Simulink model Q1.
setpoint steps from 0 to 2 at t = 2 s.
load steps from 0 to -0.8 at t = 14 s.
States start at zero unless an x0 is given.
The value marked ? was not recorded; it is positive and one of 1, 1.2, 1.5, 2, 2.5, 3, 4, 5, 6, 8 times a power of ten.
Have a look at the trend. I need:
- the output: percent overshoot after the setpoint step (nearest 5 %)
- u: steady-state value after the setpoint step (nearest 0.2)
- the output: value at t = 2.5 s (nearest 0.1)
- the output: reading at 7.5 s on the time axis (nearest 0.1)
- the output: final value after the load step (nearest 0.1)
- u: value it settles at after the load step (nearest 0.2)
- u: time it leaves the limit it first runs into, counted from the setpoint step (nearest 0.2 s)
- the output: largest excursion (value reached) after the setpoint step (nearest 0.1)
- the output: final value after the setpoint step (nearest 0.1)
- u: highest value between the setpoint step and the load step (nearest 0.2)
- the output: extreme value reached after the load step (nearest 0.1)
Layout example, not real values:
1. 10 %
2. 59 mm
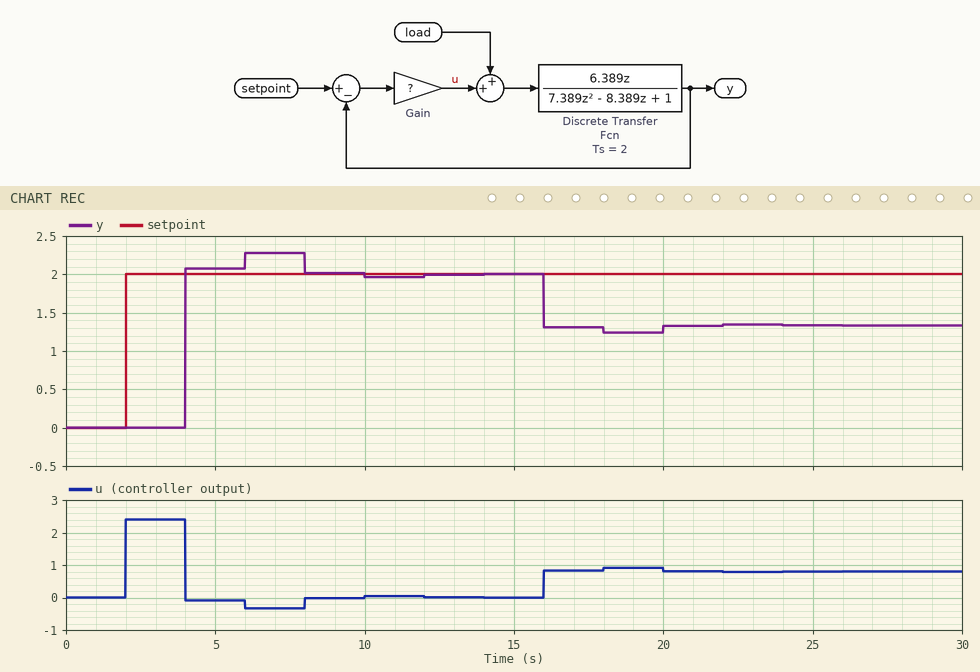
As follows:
1. 15 %
2. 0.0
3. 0.0
4. 2.3
5. 1.3
6. 0.8
7. 2.0 s
8. 2.3
9. 2.0
10. 2.4
11. 1.2
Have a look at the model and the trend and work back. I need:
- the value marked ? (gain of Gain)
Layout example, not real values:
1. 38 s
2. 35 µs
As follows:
1. 1.2
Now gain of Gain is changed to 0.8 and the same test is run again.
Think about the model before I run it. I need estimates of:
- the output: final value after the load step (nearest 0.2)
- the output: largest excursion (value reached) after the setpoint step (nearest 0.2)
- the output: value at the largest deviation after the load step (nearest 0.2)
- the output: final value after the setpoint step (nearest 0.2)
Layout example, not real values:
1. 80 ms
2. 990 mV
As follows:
1. 1.0
2. 2.0
3. 1.0
4. 2.0
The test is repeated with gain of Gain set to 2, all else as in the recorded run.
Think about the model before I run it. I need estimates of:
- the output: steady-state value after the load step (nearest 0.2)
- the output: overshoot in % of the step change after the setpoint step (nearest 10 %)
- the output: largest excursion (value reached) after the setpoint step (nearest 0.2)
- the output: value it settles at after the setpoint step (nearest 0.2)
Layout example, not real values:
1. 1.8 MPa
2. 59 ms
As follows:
1. 1.6
2. 70 %
3. 3.4
4. 2.0
